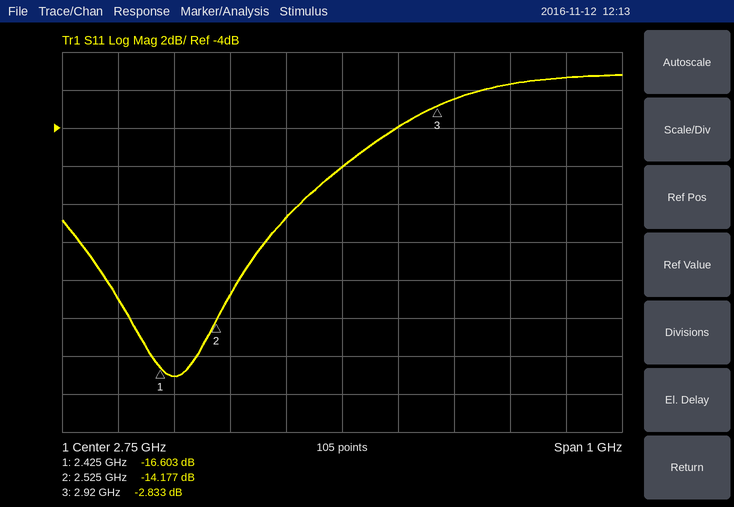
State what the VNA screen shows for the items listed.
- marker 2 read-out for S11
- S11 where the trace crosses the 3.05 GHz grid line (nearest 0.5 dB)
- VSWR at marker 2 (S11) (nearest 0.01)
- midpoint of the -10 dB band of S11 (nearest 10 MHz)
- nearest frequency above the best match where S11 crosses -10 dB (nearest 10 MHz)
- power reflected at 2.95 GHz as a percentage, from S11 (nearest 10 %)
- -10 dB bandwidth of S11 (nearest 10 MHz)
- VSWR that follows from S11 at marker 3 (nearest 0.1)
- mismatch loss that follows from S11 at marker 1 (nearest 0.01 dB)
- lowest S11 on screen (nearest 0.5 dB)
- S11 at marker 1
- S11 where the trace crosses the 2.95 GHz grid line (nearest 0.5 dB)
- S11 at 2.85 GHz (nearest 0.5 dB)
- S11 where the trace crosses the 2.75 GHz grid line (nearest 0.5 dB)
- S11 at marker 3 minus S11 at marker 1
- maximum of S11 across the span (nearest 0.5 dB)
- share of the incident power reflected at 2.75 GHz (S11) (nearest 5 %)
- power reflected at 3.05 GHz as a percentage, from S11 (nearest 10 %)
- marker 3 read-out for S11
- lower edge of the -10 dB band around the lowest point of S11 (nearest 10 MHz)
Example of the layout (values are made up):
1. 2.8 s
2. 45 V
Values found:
1. -14.177 dB
2. -1.5 dB
3. 1.49
4. 2.45 GHz
5. 2.61 GHz
6. 60 %
7. 330 MHz
8. 6.2
9. 0.10 dB
10. -17.0 dB
11. -16.603 dB
12. -2.5 dB
13. -4.0 dB
14. -6.0 dB
15. 13.770 dB
16. -1.0 dB
17. 25 %
18. 70 %
19. -2.833 dB
20. 2.28 GHz
